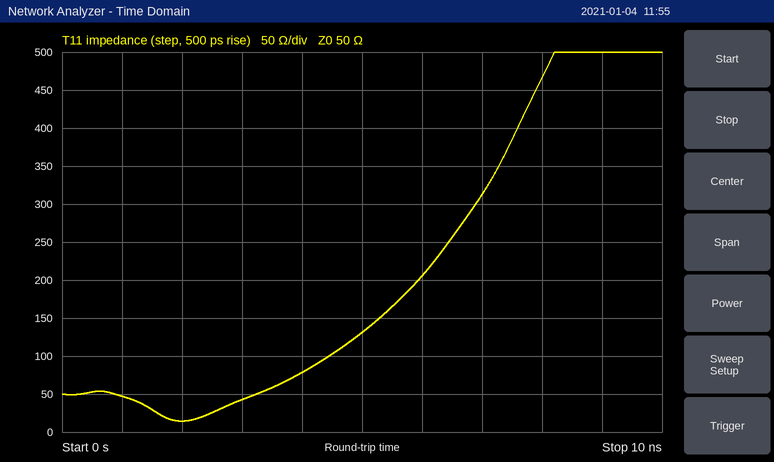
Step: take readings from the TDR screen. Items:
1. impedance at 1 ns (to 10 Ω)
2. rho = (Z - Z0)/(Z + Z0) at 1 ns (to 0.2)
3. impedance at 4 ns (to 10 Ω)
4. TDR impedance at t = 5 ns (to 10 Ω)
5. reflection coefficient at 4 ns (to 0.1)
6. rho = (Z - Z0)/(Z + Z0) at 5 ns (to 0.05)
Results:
50 Ω
0.0
80 Ω
130 Ω
+0.2
+0.45
